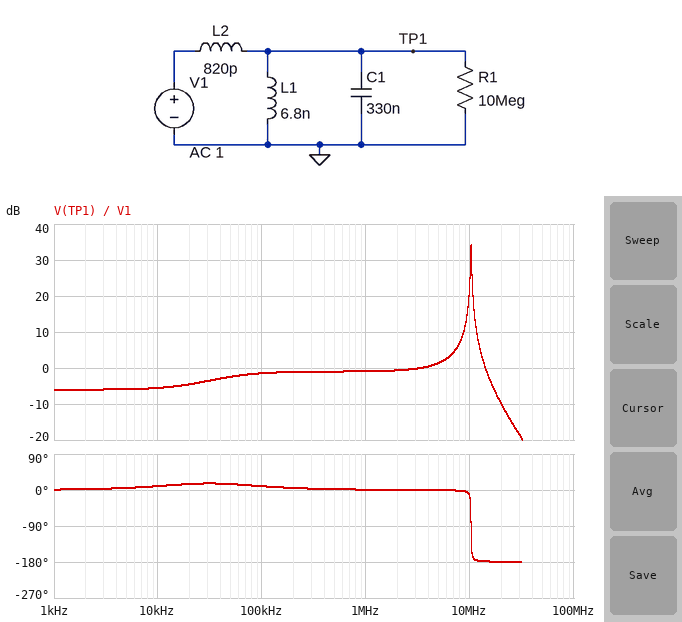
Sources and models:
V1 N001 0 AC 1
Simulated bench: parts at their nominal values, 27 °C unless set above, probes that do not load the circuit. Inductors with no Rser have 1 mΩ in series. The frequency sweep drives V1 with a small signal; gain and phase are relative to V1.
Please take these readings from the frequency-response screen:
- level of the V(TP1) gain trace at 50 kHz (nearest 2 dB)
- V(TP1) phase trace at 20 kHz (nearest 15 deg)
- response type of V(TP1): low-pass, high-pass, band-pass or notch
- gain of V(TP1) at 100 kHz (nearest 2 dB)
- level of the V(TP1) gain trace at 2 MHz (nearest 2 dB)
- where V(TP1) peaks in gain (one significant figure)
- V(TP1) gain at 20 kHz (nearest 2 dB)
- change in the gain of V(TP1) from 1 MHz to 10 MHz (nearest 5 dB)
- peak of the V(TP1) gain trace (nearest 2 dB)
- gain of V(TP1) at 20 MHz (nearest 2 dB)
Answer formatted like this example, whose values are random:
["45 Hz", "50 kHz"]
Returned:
["-2 dB", "15 deg", "band-pass", "-2 dB", "0 dB", "10 MHz", "-4 dB", "25 dB", "34 dB", "-10 dB"]
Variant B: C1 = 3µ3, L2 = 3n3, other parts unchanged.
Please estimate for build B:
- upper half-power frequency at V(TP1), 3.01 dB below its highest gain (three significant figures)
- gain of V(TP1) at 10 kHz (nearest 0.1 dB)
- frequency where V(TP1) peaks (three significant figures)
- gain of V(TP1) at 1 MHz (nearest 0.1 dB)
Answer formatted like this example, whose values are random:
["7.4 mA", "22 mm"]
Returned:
["1.88 MHz", "-5.7 dB", "1.86 MHz", "-0.5 dB"]
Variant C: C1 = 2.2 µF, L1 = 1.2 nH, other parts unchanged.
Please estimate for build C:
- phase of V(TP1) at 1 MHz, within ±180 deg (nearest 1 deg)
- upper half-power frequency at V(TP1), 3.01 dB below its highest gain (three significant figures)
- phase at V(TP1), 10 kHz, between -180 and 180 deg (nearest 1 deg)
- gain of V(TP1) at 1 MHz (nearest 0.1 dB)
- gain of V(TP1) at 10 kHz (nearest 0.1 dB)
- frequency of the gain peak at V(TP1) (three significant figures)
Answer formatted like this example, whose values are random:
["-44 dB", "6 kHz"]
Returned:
["1 deg", "4.94 MHz", "1 deg", "-4.2 dB", "-6.0 dB", "4.86 MHz"]
